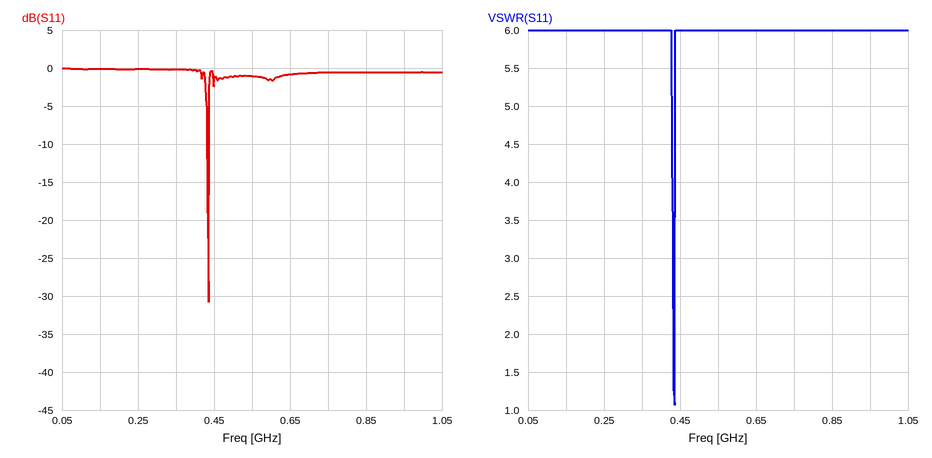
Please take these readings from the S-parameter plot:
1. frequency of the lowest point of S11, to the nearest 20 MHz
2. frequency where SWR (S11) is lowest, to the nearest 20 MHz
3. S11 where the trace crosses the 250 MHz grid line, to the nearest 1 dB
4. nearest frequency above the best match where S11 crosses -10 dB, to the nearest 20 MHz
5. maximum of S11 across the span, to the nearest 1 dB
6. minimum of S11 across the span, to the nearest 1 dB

440 MHz
440 MHz
0 dB
440 MHz
0 dB
-31 dB
